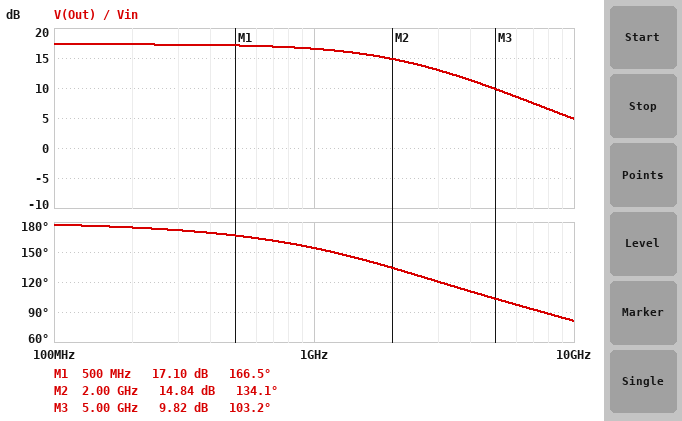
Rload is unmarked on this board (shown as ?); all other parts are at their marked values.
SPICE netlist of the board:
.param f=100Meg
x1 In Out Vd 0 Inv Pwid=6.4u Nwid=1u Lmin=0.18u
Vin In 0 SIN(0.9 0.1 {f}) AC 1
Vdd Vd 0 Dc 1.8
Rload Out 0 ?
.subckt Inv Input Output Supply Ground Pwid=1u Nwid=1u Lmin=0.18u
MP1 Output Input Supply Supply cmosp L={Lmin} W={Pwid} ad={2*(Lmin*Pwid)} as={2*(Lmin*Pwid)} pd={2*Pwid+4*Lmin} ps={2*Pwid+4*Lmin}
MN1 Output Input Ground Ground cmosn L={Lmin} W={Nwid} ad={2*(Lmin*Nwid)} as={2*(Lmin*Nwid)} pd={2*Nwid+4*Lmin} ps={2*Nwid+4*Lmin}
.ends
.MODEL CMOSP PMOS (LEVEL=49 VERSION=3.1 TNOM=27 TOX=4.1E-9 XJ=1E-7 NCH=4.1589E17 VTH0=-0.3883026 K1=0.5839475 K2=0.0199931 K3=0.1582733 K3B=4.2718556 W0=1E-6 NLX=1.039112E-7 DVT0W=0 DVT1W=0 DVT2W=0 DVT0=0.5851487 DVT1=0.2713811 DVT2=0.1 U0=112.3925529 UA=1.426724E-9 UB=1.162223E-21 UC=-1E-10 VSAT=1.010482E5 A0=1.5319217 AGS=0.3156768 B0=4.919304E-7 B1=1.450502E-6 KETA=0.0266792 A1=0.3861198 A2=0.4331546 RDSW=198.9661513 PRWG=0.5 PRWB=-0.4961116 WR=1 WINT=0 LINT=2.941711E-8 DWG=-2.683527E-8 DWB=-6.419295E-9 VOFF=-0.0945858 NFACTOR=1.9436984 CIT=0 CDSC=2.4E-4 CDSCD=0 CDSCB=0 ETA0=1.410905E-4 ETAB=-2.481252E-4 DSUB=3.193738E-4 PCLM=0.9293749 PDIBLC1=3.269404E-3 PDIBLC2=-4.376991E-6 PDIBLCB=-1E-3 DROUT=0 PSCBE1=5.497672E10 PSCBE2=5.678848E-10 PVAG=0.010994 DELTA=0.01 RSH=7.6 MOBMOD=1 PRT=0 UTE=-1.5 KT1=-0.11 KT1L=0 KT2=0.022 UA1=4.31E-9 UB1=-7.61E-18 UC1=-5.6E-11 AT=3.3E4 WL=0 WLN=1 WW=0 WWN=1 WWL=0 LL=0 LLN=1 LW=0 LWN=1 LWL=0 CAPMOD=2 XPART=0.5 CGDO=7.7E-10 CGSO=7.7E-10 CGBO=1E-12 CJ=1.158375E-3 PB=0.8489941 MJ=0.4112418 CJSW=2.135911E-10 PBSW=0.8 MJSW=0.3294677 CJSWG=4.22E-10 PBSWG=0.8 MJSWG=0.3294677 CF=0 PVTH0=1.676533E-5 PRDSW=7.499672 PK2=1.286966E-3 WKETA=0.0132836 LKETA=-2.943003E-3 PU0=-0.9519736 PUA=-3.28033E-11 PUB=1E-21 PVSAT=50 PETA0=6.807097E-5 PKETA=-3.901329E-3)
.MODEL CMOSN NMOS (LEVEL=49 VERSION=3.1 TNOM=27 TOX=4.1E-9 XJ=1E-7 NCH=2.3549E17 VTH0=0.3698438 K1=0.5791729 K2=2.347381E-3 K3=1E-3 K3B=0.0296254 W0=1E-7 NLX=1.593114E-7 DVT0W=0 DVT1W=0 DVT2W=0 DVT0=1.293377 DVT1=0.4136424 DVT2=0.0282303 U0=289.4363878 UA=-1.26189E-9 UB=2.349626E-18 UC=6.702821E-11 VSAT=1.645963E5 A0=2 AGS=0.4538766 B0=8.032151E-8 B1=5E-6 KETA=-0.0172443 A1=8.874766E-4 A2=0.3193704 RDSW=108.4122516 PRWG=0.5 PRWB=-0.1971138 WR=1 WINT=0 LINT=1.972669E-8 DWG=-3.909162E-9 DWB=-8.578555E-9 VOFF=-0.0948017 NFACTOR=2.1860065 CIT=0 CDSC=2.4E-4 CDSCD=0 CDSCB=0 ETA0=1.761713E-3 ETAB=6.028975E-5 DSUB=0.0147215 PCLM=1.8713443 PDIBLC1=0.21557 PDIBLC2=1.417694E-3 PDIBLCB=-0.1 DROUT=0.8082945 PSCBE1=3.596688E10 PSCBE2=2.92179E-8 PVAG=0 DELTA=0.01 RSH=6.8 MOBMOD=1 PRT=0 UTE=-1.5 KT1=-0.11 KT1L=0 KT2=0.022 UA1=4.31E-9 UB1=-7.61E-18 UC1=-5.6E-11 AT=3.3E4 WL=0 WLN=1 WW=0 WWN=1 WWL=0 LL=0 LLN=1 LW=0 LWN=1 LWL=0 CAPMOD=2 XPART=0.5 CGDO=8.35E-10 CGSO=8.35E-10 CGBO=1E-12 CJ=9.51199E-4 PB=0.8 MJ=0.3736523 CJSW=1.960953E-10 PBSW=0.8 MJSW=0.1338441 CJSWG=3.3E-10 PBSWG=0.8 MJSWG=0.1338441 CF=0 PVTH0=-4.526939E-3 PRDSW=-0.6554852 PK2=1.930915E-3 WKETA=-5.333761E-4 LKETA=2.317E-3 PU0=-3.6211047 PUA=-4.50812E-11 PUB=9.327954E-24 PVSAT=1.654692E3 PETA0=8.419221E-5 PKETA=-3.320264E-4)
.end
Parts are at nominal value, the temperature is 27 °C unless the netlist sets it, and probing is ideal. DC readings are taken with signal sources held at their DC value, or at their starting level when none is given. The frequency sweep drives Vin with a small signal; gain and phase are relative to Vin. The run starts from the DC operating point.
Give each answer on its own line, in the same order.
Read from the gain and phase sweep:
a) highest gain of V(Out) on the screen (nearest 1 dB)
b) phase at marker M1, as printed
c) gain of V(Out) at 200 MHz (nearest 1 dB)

17 dB
166.5 deg
17 dB
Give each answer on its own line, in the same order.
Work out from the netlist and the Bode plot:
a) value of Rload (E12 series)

27 kΩ
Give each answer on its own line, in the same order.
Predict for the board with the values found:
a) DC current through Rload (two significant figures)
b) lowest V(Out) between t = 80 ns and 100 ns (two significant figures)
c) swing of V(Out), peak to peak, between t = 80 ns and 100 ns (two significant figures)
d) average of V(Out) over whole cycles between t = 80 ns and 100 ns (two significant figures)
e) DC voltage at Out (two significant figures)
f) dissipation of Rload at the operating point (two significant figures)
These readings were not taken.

53 µA
240 mV
1.4 V
1.1 V
1.4 V
75 µW
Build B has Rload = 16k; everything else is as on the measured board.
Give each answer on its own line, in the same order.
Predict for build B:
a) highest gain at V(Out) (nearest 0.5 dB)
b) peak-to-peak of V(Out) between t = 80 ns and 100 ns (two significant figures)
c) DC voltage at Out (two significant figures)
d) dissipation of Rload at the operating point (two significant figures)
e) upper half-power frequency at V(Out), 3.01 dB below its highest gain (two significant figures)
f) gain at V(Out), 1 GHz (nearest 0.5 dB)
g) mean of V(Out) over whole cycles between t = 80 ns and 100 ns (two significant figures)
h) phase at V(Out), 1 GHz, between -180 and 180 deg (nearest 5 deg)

20.5 dB
1.4 V
1.2 V
89 µW
1.7 GHz
19.5 dB
1.0 V
150 deg
